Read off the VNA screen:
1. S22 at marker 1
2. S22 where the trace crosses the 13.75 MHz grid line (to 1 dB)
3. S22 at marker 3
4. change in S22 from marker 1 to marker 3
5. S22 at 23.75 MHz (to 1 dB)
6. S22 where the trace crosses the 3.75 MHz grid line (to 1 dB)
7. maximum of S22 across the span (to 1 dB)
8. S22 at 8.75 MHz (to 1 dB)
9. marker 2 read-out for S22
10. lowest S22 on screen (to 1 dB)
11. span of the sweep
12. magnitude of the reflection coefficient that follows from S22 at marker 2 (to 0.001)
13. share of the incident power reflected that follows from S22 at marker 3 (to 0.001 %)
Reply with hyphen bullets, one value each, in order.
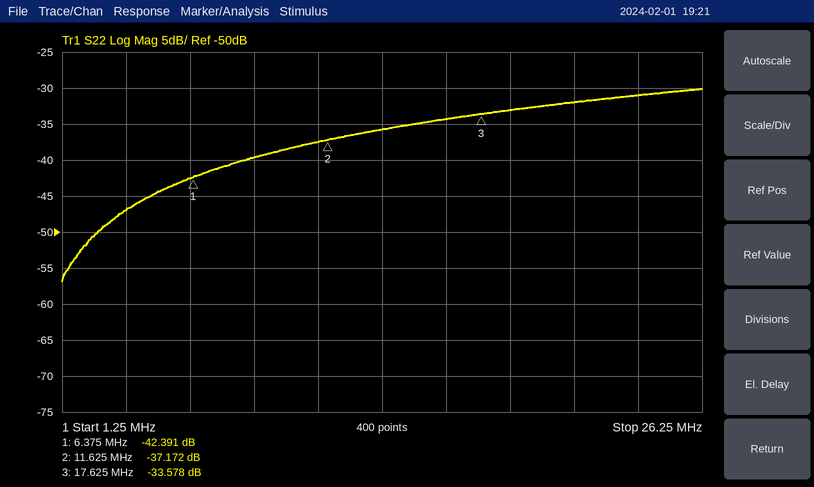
- -42.391 dB
- -36 dB
- -33.578 dB
- 8.813 dB
- -31 dB
- -47 dB
- -30 dB
- -40 dB
- -37.172 dB
- -57 dB
- 25 MHz
- 0.014
- 0.044 %
